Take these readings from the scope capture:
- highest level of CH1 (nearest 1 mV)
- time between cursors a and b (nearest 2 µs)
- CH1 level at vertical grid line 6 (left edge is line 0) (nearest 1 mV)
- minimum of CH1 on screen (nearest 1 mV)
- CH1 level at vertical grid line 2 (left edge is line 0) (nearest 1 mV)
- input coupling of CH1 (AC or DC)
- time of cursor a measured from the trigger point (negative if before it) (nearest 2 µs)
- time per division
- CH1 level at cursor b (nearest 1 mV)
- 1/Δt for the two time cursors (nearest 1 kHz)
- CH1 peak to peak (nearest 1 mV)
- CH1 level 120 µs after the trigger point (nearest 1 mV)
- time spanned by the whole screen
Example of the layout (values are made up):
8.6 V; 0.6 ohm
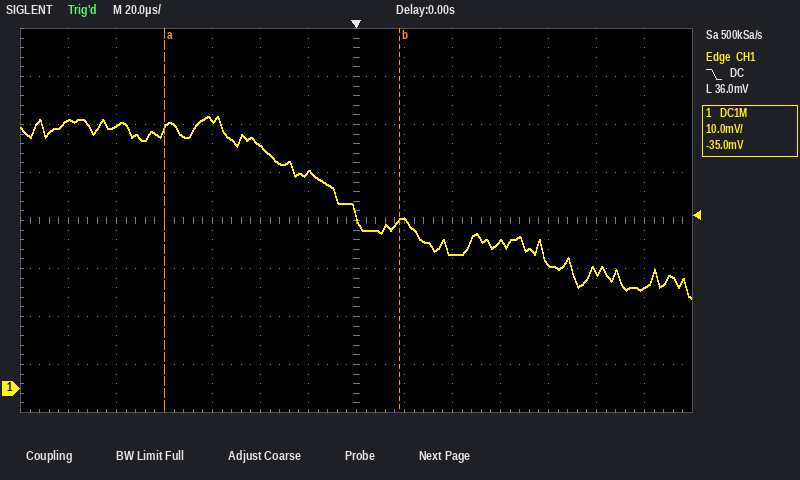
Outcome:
57 mV; 98 µs; 45 mV; 19 mV; 55 mV; DC; -80 µs; 20 µs; 35 mV; 10 kHz; 38 mV; 21 mV; 280 µs
